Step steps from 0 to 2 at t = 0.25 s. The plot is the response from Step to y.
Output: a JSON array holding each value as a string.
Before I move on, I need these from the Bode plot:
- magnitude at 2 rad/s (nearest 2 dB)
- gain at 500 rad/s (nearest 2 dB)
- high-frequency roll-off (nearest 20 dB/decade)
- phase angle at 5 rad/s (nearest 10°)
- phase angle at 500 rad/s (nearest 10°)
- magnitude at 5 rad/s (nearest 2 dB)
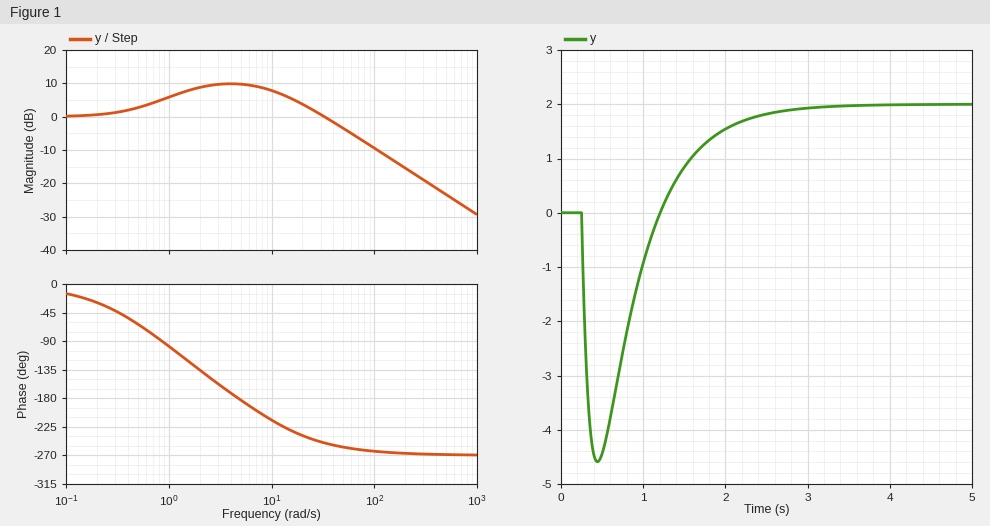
["8 dB", "-24 dB", "-20 dB/decade", "-180°", "-270°", "10 dB"]
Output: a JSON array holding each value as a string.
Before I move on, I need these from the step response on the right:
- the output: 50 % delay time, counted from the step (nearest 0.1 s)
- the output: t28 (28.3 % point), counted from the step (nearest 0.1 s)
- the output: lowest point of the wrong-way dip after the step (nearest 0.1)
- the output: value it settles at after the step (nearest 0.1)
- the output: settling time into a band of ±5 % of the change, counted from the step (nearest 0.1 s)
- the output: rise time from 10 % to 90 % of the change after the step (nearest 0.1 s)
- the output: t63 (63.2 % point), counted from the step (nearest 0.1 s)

["1.3 s", "1.1 s", "-4.6", "2.0", "2.6 s", "1.2 s", "1.5 s"]
